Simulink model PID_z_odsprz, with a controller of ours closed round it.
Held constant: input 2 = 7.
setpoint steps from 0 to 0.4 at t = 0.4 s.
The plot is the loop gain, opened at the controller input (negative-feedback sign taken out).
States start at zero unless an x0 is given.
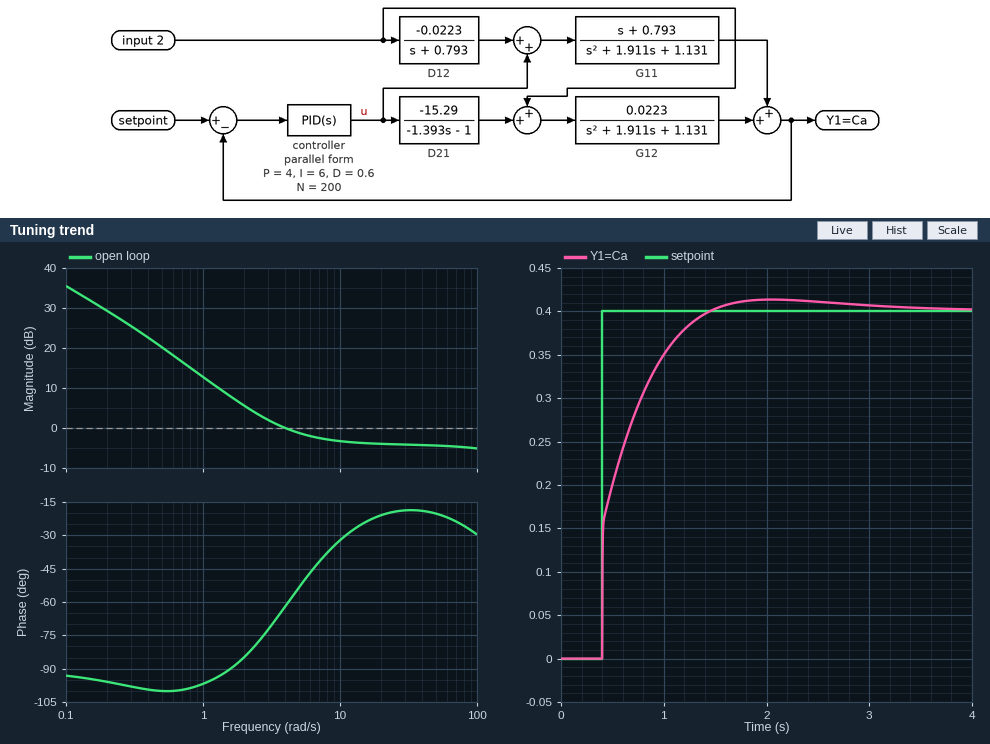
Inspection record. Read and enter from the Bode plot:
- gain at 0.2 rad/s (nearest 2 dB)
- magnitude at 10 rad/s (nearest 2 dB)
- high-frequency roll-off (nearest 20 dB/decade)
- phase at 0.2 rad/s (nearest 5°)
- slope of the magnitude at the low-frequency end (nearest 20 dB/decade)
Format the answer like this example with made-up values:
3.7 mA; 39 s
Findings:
30 dB; -4 dB; 0 dB/decade; -95°; -20 dB/decade
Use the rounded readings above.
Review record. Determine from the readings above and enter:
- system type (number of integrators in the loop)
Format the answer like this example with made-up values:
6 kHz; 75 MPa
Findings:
1
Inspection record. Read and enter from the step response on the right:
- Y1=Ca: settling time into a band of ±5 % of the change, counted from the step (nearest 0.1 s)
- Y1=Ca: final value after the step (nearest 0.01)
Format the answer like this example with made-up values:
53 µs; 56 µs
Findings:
0.8 s; 0.40
